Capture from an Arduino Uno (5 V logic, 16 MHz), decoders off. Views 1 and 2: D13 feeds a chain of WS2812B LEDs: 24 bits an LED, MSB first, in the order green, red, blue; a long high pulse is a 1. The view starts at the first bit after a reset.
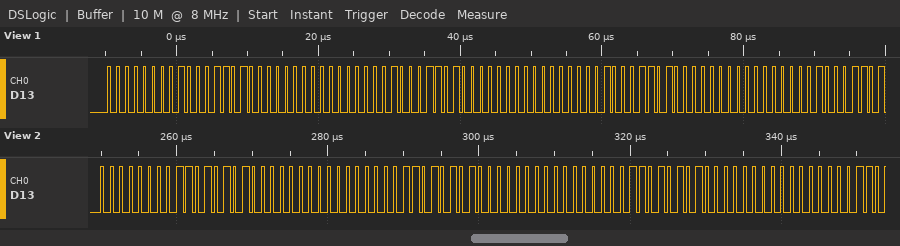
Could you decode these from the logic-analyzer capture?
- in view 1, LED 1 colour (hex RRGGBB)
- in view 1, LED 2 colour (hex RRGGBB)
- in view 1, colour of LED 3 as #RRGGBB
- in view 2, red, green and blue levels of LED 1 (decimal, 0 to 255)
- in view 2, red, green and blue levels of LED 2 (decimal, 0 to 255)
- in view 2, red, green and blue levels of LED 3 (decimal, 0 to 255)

#8D0000
#8D0000
#8D0000
213, 0, 0
213, 0, 0
213, 0, 0
